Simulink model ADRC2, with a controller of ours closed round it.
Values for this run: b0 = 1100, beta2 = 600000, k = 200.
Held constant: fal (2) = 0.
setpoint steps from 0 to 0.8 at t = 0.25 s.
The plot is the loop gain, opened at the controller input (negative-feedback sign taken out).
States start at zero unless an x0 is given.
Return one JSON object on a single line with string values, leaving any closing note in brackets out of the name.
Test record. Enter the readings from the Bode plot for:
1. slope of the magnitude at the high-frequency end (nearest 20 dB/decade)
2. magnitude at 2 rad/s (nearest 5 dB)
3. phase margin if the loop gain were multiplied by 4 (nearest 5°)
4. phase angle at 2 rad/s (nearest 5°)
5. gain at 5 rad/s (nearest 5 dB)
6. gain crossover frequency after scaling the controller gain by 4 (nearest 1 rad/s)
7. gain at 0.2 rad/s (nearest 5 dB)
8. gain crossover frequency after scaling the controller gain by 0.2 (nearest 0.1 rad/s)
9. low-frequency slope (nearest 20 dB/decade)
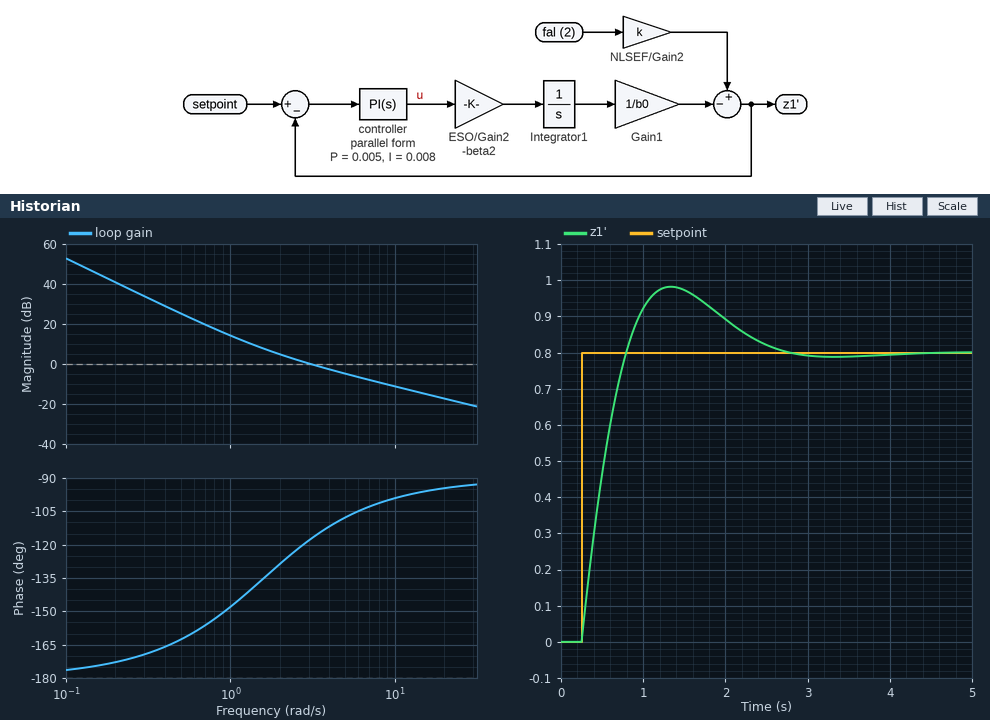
{"slope of the magnitude at the high-frequency end": "-20 dB/decade", "magnitude at 2 rad/s": "5 dB", "phase margin if the loop gain were multiplied by 4": "80°", "phase angle at 2 rad/s": "-130°", "gain at 5 rad/s": "-5 dB", "gain crossover frequency after scaling the controller gain by 4": "11 rad/s", "gain at 0.2 rad/s": "40 dB", "gain crossover frequency after scaling the controller gain by 0.2": "1.0 rad/s", "low-frequency slope": "-40 dB/decade"}
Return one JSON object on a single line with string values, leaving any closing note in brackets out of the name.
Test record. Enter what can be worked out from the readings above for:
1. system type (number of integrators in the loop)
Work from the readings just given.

{"system type": "2"}
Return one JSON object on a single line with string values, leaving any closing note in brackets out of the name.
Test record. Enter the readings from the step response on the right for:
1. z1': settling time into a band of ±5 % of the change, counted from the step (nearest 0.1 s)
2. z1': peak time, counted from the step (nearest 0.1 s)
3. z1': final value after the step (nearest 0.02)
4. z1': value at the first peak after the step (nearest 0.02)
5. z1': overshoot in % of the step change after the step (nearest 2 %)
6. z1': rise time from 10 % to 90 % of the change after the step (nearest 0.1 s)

{"z1': settling time into a band of ±5 % of the change, counted from the step": "2.1 s", "z1': peak time, counted from the step": "1.1 s", "z1': final value after the step": "0.80", "z1': value at the first peak after the step": "0.98", "z1': overshoot in % of the step change after the step": "22 %", "z1': rise time from 10 % to 90 % of the change after the step": "0.4 s"}
